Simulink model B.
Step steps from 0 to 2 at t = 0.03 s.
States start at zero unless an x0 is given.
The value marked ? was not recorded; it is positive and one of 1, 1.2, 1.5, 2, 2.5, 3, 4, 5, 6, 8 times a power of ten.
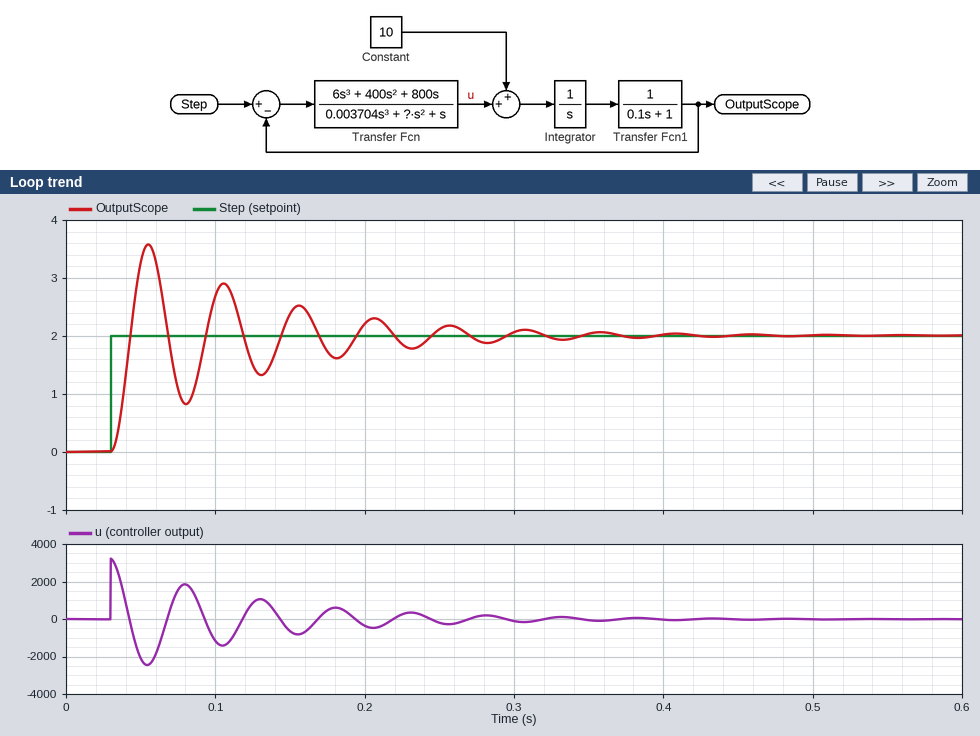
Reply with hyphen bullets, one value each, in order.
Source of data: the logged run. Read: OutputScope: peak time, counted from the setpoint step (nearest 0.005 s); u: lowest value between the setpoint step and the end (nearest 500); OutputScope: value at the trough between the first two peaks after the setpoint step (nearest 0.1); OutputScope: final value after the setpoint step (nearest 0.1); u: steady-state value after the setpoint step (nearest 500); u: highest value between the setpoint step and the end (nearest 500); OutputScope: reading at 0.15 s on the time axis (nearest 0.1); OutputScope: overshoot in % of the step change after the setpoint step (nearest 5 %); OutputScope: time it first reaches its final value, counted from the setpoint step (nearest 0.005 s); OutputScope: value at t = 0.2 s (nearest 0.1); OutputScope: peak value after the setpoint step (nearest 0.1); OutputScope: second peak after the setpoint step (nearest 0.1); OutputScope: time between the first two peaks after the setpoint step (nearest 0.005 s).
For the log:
- 0.025 s
- -2500
- 0.8
- 2.0
- 0
- 3000
- 2.4
- 80 %
- 0.015 s
- 2.2
- 3.6
- 2.9
- 0.050 s
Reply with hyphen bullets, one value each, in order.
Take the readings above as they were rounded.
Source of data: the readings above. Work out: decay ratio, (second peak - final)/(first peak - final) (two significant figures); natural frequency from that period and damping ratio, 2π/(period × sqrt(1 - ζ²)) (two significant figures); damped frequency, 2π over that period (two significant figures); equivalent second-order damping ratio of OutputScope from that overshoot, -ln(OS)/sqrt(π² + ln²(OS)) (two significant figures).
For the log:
- 0.56
- 130 rad/s
- 130 rad/s
- 0.071
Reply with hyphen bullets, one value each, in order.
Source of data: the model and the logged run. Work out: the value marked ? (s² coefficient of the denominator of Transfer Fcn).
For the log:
- 0.3
